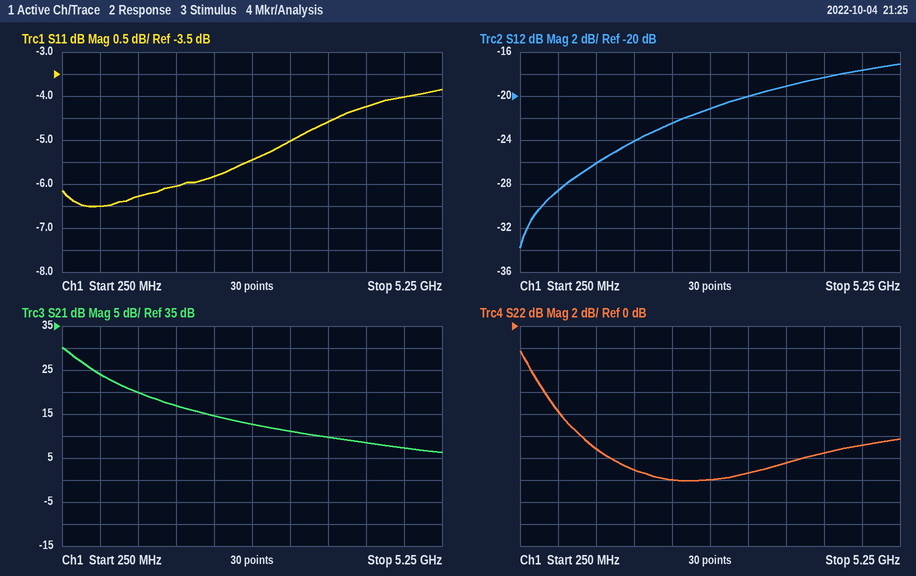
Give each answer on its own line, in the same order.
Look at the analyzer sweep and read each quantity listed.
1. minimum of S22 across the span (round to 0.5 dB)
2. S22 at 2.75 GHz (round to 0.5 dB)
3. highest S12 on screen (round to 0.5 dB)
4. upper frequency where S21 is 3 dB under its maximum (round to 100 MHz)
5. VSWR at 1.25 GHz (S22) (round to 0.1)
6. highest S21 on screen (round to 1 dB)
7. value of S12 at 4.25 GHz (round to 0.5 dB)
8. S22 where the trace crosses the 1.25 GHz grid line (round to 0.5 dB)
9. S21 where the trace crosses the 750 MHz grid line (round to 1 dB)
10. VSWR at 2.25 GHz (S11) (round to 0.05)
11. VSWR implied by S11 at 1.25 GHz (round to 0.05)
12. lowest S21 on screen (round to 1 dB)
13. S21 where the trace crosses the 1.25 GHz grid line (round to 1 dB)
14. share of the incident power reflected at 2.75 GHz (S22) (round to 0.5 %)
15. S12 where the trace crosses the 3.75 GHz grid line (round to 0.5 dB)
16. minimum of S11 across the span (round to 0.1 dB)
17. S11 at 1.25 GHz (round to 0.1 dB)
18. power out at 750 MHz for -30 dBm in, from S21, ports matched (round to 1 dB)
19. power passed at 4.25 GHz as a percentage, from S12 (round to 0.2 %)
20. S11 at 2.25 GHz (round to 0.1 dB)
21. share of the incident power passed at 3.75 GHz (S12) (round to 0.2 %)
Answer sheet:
-14.0 dB
-14.0 dB
-17.0 dB
500 MHz
1.8
30 dB
-18.5 dB
-11.0 dB
24 dB
3.10
2.90
6 dB
20 dB
4.0 %
-19.0 dB
-6.5 dB
-6.3 dB
-6 dBm
1.4 %
-5.8 dB
1.2 %
